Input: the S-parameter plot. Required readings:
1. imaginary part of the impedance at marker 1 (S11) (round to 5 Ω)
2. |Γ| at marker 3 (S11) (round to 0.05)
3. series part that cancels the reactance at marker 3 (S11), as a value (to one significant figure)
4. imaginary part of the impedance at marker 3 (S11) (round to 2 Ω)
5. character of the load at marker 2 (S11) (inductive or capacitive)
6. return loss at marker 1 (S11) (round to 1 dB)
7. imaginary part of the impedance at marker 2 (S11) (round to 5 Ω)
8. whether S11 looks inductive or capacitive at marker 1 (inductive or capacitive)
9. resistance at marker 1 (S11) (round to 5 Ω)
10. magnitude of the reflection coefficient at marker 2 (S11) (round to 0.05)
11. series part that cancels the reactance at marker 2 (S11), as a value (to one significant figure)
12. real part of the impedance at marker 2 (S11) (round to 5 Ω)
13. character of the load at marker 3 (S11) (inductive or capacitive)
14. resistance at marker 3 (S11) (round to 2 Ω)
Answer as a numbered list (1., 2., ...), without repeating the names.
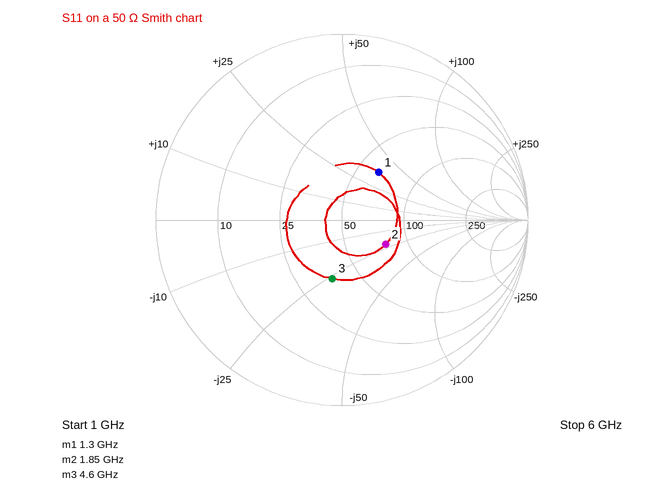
1. +35 Ω
2. 0.30
3. 900 pH
4. -26 Ω
5. capacitive
6. 10 dB
7. -20 Ω
8. inductive
9. 65 Ω
10. 0.25
11. 2 nH
12. 75 Ω
13. capacitive
14. 38 Ω
